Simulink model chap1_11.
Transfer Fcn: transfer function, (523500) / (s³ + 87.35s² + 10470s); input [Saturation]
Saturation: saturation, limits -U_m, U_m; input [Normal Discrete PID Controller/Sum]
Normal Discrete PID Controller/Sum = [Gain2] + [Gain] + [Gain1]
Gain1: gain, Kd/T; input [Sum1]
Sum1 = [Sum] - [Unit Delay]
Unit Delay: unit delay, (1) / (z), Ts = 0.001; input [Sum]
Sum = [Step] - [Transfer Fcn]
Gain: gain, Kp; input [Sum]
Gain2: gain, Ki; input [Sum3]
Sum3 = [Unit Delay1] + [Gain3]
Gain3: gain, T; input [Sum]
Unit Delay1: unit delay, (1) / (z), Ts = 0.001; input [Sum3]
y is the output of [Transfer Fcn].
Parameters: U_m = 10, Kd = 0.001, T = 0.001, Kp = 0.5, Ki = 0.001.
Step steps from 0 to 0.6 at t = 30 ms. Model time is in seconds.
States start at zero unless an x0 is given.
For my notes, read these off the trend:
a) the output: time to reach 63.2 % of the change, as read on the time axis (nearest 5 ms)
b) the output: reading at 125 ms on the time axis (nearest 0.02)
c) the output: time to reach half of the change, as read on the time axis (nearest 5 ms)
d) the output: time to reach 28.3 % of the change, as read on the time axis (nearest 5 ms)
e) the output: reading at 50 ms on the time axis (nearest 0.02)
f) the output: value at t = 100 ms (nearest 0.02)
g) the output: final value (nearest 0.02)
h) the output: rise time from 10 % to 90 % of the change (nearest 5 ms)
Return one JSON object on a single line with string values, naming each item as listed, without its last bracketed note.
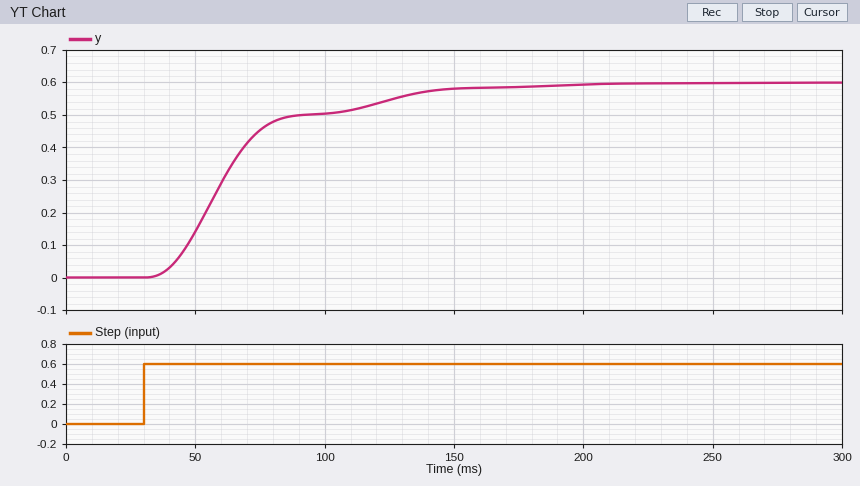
{"the output: time to reach 63.2 % of the change, as read on the time axis": "65 ms", "the output: reading at 125 ms on the time axis": "0.54", "the output: time to reach half of the change, as read on the time axis": "60 ms", "the output: time to reach 28.3 % of the change, as read on the time axis": "50 ms", "the output: reading at 50 ms on the time axis": "0.14", "the output: value at t = 100 ms": "0.50", "the output: final value": "0.60", "the output: rise time from 10 % to 90 % of the change": "80 ms"}
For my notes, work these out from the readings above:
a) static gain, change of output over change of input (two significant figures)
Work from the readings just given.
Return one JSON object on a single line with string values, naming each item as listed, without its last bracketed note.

{"static gain, change of output over change of input": "1.0"}
